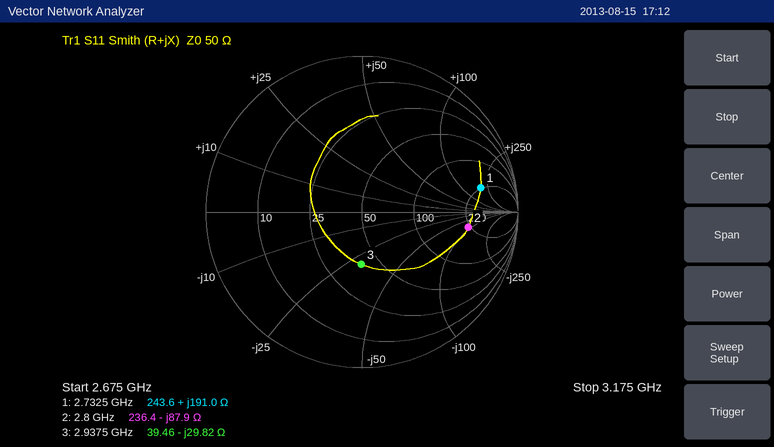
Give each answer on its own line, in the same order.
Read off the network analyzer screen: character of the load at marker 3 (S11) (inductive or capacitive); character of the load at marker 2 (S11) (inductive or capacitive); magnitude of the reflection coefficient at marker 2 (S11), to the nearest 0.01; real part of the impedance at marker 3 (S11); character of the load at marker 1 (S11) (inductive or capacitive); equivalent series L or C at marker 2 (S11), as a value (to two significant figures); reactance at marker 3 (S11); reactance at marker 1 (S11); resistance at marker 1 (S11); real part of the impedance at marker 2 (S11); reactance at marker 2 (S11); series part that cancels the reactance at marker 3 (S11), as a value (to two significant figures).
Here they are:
capacitive
capacitive
0.69
39.46 Ω
inductive
650 fF
-29.82 Ω
+191.0 Ω
243.6 Ω
236.4 Ω
-87.9 Ω
1.6 nH
